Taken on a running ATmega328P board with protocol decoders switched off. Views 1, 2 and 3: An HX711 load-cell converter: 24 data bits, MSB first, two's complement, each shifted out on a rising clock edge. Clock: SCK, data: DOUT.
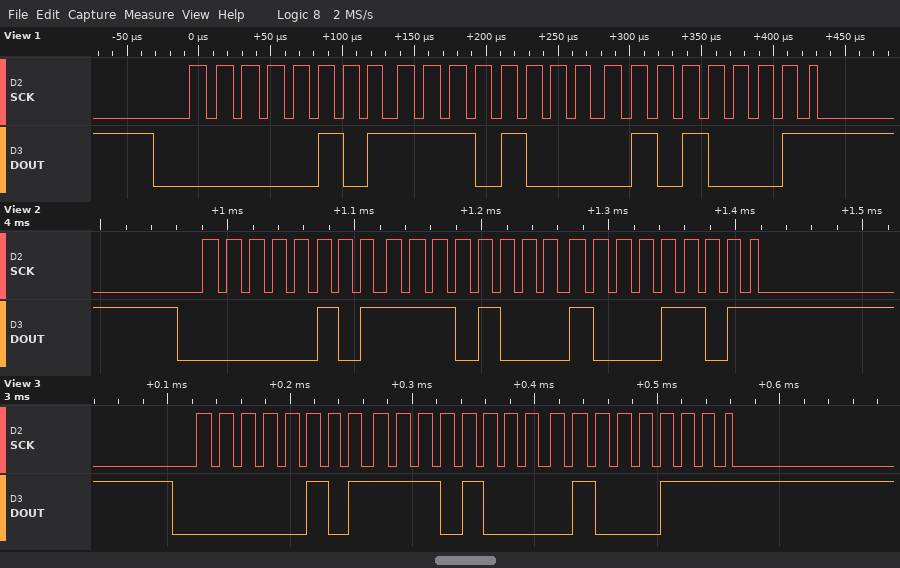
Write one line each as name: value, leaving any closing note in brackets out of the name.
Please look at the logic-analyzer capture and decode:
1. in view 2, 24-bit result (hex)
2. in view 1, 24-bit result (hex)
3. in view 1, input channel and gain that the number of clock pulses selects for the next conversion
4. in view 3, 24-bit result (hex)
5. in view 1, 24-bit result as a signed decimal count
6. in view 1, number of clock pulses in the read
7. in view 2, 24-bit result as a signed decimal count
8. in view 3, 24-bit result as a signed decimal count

in view 2, 24-bit result: 0x05E88D
in view 1, 24-bit result: 0x05E851
in view 1, input channel and gain that the number of clock pulses selects for the next conversion: channel A, gain 128
in view 3, 24-bit result: 0x05E847
in view 1, 24-bit result as a signed decimal count: 387153
in view 1, number of clock pulses in the read: 25
in view 2, 24-bit result as a signed decimal count: 387213
in view 3, 24-bit result as a signed decimal count: 387143
